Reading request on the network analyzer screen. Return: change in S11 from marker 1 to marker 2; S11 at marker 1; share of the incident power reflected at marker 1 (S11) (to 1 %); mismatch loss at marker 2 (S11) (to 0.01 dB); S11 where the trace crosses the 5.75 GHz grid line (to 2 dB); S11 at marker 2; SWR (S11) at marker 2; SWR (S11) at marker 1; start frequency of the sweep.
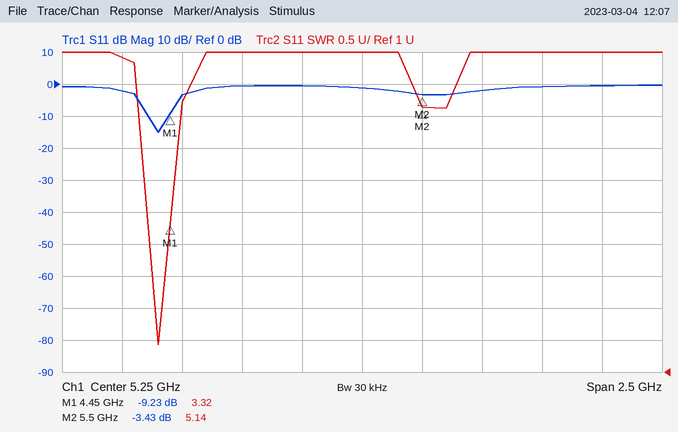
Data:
5.80 dB
-9.23 dB
12 %
2.63 dB
-2 dB
-3.43 dB
5.14
3.32
4 GHz
